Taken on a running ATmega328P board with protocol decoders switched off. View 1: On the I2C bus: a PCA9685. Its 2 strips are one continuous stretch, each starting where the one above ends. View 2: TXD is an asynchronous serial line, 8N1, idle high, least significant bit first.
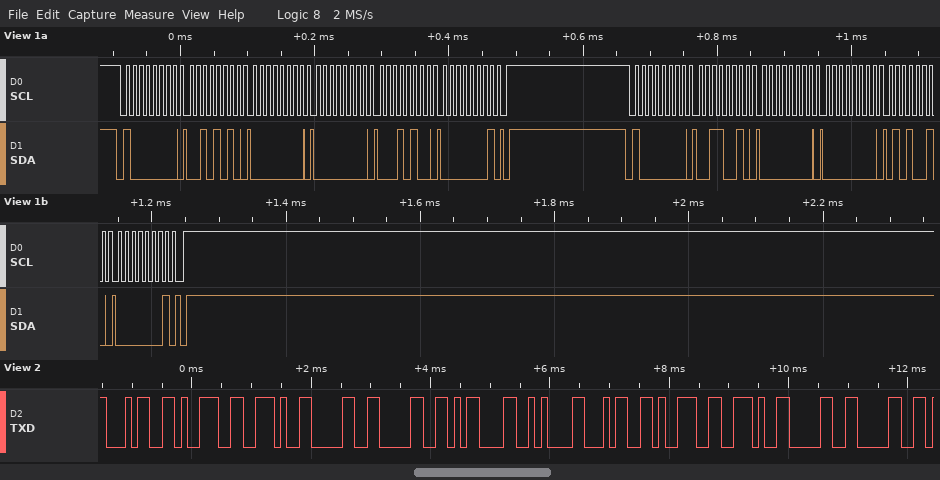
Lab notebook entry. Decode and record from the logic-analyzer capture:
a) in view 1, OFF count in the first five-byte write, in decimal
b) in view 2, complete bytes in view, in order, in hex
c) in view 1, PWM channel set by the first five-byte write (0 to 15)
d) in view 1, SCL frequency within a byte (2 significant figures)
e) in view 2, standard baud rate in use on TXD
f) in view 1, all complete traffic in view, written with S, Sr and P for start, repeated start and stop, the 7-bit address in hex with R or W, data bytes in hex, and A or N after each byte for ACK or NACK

276
0x34 0x39 0x2E 0x30 0x30 0x0D 0x0A 0x34 0x39 0x2E 0x30 0x30
9
100 kHz
9600 baud
S 40W A 2A A 00 A 00 A 14 A 01 A P S 40W A 32 A 00 A 00 A 52 A 01 A P
